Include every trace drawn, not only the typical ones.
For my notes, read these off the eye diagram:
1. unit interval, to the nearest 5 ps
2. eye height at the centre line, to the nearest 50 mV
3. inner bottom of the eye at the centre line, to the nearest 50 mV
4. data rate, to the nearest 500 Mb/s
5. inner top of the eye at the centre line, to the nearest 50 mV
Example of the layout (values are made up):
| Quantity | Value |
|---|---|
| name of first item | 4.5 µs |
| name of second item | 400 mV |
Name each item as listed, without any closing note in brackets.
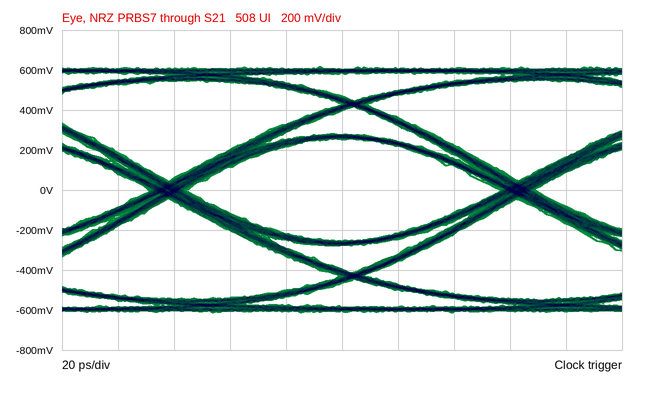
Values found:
| Quantity | Value |
|---|---|
| unit interval, to the nearest 5 ps | 125 ps |
| eye height at the centre line, to the nearest 50 mV | 500 mV |
| inner bottom of the eye at the centre line, to the nearest 50 mV | -250 mV |
| data rate, to the nearest 500 Mb/s | 8.0 Gb/s |
| inner top of the eye at the centre line, to the nearest 50 mV | 250 mV |
